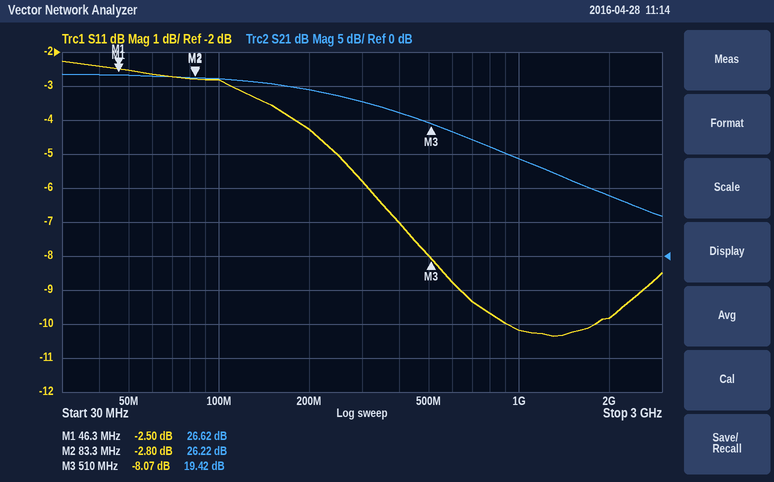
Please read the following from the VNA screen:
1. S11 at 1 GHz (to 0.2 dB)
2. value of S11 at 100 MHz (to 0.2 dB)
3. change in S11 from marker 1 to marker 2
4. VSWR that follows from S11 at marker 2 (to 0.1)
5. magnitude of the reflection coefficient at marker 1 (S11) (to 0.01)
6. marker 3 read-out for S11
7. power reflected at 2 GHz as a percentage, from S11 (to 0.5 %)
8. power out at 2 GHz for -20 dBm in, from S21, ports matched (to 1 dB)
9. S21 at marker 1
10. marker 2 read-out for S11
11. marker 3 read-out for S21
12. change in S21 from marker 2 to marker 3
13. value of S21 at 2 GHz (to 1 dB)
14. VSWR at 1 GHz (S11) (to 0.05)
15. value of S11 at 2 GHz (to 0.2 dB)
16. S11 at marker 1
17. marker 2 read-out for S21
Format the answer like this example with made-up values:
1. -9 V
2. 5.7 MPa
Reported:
1. -10.2 dB
2. -2.8 dB
3. -0.30 dB
4. 6.3
5. 0.75
6. -8.07 dB
7. 10.5 %
8. -11 dBm
9. 26.62 dB
10. -2.80 dB
11. 19.42 dB
12. -6.80 dB
13. 9 dB
14. 1.90
15. -9.8 dB
16. -2.50 dB
17. 26.22 dB
